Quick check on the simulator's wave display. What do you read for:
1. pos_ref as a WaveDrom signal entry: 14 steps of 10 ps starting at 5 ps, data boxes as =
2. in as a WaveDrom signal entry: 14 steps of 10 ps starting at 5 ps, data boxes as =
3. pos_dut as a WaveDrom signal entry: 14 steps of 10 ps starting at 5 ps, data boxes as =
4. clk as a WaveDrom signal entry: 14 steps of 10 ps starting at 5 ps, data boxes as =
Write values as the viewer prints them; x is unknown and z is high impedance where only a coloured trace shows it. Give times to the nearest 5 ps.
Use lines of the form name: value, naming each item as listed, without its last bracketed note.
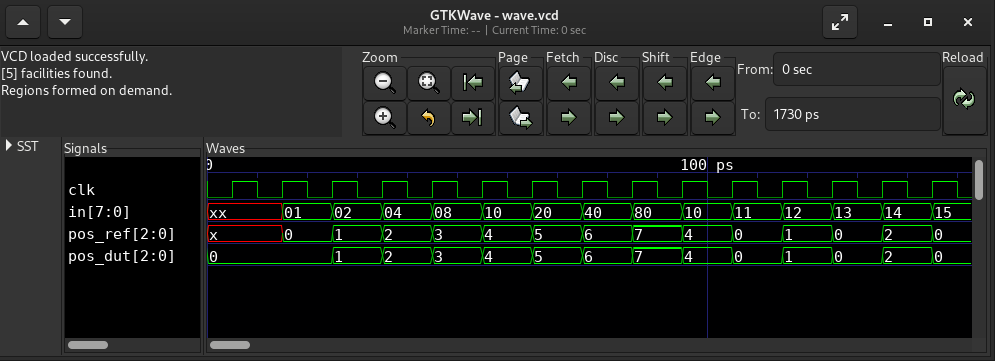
pos_ref as a WaveDrom signal entry: 14 steps of 10 ps starting at 5 ps, data boxes as =: {name: 'pos_ref', wave: 'x=============', data: '0 1 2 3 4 5 6 7 4 0 1 0 2'}
in as a WaveDrom signal entry: 14 steps of 10 ps starting at 5 ps, data boxes as =: {name: 'in', wave: 'x=============', data: '01 02 04 08 10 20 40 80 10 11 12 13 14'}
pos_dut as a WaveDrom signal entry: 14 steps of 10 ps starting at 5 ps, data boxes as =: {name: 'pos_dut', wave: '=.============', data: '0 1 2 3 4 5 6 7 4 0 1 0 2'}
clk as a WaveDrom signal entry: 14 steps of 10 ps starting at 5 ps, data boxes as =: {name: 'clk', wave: 'p.............'}
